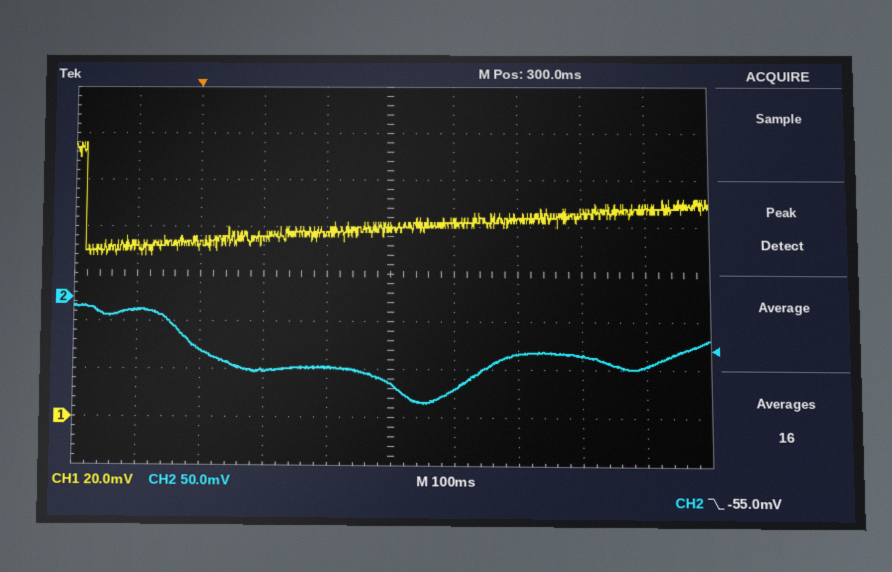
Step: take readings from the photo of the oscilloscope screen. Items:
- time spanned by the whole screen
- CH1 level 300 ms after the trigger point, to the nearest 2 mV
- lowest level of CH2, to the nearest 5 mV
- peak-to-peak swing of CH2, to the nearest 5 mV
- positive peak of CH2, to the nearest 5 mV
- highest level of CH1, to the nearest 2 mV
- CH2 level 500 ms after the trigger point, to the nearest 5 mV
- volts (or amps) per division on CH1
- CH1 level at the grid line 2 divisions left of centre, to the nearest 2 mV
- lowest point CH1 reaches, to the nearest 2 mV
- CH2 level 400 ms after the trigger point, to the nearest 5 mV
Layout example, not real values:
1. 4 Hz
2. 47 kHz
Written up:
1. 1 s
2. 80 mV
3. -110 mV
4. 100 mV
5. -10 mV
6. 116 mV
7. -60 mV
8. 20 mV
9. 74 mV
10. 68 mV
11. -95 mV
